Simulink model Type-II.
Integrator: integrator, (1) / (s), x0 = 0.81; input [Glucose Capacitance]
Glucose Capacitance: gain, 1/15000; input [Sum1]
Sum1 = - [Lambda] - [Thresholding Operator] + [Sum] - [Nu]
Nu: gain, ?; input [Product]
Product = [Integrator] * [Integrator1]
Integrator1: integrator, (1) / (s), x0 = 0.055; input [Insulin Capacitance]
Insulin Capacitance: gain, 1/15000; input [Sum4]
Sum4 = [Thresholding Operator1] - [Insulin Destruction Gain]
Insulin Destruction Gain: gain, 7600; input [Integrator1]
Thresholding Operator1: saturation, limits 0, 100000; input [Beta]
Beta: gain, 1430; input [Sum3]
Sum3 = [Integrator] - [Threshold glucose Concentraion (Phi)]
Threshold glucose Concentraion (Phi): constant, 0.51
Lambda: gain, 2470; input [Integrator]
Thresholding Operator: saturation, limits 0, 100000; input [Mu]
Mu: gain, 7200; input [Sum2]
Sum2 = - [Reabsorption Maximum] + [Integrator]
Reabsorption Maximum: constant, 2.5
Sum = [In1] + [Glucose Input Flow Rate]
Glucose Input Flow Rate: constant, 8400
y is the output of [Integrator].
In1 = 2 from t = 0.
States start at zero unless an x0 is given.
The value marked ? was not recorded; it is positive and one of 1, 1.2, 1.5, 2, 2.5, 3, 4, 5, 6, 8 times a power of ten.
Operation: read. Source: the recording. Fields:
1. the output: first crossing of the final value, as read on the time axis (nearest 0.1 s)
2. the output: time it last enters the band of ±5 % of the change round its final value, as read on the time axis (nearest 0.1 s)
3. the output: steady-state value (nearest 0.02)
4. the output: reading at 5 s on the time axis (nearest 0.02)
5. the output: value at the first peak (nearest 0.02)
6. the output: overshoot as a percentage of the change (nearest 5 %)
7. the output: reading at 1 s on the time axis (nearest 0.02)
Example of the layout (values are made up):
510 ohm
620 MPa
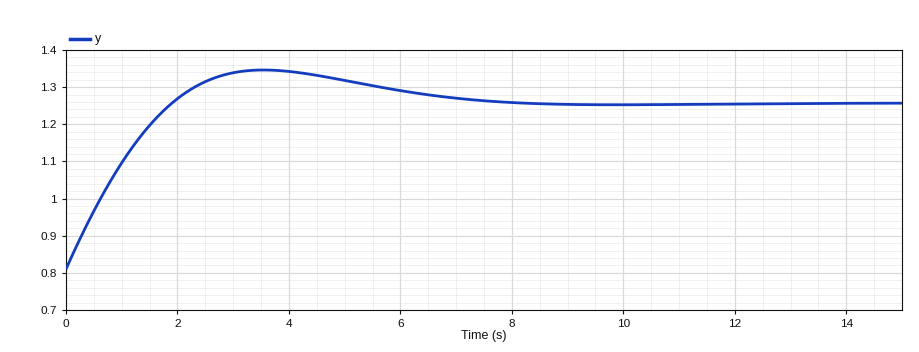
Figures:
1.9 s
6.5 s
1.26
1.32
1.34
20 %
1.10
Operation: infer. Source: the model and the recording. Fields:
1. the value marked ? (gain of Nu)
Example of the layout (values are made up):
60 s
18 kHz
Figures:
30000
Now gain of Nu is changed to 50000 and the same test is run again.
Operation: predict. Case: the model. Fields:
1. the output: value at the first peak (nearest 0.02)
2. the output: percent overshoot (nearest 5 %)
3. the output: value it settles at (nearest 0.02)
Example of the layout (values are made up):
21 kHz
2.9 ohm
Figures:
1.16
30 %
1.08
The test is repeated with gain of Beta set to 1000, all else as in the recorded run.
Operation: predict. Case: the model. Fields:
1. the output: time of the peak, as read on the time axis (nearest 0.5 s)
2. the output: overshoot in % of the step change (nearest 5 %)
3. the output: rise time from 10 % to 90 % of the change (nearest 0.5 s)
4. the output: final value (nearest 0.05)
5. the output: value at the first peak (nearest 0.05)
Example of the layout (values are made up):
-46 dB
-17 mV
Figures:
4.5 s
10 %
2.0 s
1.40
1.45
